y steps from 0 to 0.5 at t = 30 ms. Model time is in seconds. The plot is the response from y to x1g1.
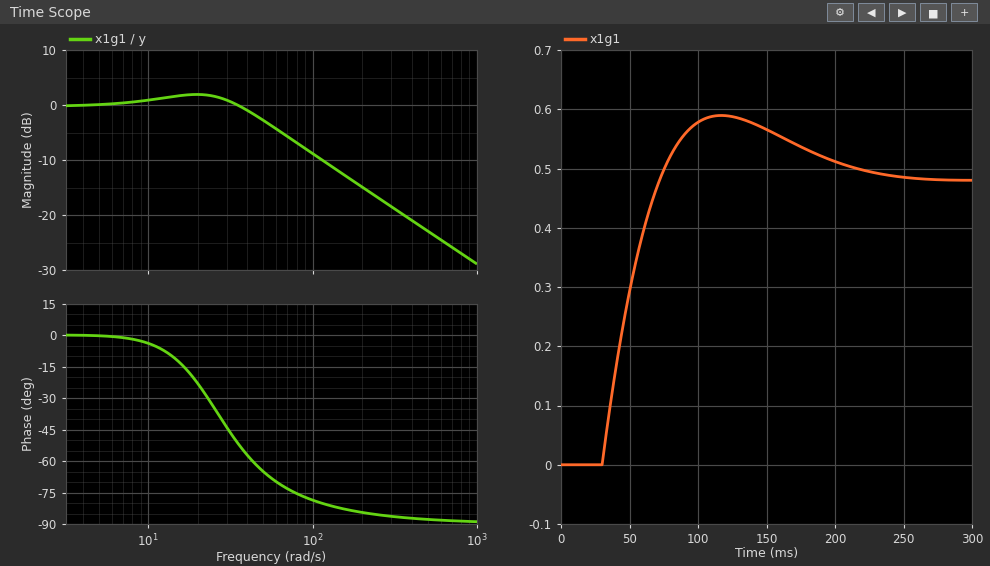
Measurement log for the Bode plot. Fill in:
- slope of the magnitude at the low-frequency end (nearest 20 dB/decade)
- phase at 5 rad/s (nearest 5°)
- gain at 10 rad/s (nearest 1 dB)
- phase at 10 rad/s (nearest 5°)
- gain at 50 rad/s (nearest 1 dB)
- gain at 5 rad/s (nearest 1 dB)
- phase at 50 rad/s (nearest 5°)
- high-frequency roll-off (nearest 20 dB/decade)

0 dB/decade
0°
1 dB
-5°
-3 dB
0 dB
-65°
-20 dB/decade
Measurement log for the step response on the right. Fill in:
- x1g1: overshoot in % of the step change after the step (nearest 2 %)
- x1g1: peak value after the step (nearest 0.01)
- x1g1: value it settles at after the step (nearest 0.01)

22 %
0.59
0.48
